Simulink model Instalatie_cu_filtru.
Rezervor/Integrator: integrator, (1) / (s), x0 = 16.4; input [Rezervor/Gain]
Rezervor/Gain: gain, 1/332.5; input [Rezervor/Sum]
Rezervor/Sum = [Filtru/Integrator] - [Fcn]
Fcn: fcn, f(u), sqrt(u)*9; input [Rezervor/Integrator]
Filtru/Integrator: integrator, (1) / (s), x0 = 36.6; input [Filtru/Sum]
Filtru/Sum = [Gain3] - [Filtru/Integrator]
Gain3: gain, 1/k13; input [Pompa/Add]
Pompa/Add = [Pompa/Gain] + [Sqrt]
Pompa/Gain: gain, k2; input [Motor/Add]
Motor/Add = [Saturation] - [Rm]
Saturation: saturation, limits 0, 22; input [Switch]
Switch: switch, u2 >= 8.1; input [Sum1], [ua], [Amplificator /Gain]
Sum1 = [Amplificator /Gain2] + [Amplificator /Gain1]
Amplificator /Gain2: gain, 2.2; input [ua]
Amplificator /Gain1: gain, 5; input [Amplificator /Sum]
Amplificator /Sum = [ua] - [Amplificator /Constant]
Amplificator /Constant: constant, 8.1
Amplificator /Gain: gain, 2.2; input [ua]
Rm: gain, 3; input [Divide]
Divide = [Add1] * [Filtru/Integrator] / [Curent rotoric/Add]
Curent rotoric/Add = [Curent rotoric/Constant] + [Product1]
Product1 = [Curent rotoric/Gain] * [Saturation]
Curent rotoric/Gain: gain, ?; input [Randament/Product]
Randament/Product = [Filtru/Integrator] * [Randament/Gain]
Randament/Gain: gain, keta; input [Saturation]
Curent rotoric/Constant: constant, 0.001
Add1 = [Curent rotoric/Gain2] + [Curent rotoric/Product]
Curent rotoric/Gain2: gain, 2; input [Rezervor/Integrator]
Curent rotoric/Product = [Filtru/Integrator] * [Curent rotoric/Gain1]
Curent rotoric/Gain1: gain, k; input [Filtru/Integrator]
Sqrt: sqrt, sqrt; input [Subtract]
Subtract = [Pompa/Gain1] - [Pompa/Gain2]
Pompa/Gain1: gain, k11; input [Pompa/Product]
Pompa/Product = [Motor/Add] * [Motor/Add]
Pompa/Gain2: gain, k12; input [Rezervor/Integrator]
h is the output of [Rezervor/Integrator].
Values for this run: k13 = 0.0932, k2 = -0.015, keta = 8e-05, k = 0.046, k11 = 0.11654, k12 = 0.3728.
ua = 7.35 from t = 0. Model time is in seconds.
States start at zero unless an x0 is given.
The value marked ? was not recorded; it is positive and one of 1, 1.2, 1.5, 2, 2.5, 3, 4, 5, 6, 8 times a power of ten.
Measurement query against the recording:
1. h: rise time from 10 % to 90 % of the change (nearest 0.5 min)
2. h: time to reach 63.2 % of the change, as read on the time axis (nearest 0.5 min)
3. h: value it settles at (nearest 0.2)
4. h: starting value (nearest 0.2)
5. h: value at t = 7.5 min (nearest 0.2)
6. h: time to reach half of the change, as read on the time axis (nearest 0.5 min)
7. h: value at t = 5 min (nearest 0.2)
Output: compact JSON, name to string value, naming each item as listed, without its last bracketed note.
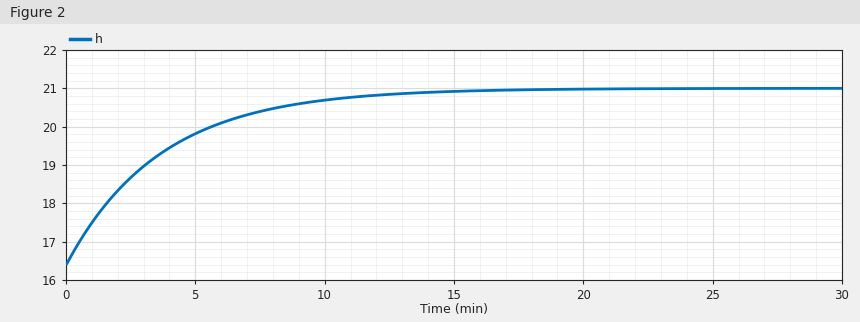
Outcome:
{"h: rise time from 10 % to 90 % of the change": "8.0 min", "h: time to reach 63.2 % of the change, as read on the time axis": "3.5 min", "h: value it settles at": "21.0", "h: starting value": "16.4", "h: value at t = 7.5 min": "20.4", "h: time to reach half of the change, as read on the time axis": "2.5 min", "h: value at t = 5 min": "19.8"}
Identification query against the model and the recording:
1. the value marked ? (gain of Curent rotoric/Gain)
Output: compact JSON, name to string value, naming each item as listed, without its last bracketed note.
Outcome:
{"the value marked ?": "10000"}
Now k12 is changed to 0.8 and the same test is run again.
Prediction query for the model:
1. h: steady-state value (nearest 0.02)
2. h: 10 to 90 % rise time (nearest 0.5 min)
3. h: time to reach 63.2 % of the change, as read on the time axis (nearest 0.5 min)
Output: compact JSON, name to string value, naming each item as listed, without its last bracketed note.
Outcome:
{"h: steady-state value": "16.06", "h: 10 to 90 % rise time": "5.5 min", "h: time to reach 63.2 % of the change, as read on the time axis": "2.5 min"}
